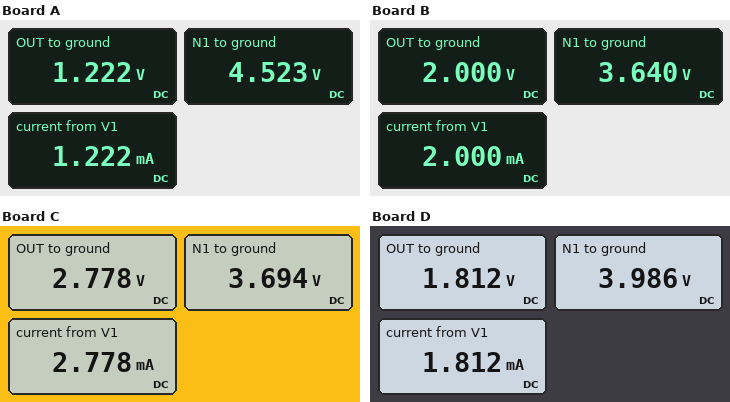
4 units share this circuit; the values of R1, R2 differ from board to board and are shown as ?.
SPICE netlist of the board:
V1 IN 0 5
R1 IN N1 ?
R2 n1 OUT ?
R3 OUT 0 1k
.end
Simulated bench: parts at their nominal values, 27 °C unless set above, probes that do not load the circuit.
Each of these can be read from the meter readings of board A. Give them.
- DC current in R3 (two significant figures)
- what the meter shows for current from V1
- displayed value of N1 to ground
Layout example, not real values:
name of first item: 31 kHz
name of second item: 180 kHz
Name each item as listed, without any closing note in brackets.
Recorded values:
DC current in R3: 1.2 mA
what the meter shows for current from V1: 1.222 mA
displayed value of N1 to ground: 4.523 V
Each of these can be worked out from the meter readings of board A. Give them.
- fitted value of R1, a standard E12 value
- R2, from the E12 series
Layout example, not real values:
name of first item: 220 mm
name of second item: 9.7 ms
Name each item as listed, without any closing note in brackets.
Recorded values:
fitted value of R1, a standard E12 value: 390 Ω
R2, from the E12 series: 2.7 kΩ
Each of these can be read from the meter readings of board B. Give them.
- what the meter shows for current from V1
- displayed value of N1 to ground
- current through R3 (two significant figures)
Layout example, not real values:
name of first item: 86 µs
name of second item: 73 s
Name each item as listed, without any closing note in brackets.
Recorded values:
what the meter shows for current from V1: 2.000 mA
displayed value of N1 to ground: 3.640 V
current through R3: 2.0 mA
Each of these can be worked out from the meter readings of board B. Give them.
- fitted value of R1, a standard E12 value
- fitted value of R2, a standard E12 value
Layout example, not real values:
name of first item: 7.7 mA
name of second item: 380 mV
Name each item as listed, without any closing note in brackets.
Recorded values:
fitted value of R1, a standard E12 value: 680 Ω
fitted value of R2, a standard E12 value: 820 Ω
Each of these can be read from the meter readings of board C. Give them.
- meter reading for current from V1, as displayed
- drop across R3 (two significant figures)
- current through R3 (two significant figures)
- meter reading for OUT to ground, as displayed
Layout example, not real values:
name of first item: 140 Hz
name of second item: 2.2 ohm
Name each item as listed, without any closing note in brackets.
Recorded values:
meter reading for current from V1, as displayed: 2.778 mA
drop across R3: 2.8 V
current through R3: 2.8 mA
meter reading for OUT to ground, as displayed: 2.778 V
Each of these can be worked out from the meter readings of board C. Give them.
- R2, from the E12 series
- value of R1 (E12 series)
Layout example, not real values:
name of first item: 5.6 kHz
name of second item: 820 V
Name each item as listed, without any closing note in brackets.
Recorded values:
R2, from the E12 series: 330 Ω
value of R1: 470 Ω
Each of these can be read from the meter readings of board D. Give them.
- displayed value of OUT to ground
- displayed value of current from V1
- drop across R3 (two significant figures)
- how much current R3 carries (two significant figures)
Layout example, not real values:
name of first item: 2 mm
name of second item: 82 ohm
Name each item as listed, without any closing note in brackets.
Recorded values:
displayed value of OUT to ground: 1.812 V
displayed value of current from V1: 1.812 mA
drop across R3: 1.8 V
how much current R3 carries: 1.8 mA
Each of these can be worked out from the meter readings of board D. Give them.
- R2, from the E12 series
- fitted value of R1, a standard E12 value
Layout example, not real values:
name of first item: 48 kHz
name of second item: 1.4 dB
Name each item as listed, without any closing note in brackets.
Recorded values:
R2, from the E12 series: 1.2 kΩ
fitted value of R1, a standard E12 value: 560 Ω
